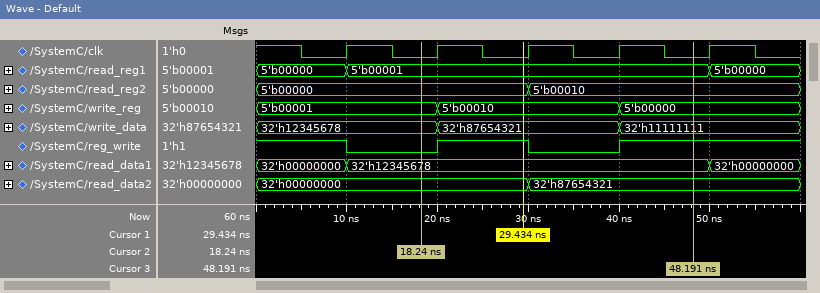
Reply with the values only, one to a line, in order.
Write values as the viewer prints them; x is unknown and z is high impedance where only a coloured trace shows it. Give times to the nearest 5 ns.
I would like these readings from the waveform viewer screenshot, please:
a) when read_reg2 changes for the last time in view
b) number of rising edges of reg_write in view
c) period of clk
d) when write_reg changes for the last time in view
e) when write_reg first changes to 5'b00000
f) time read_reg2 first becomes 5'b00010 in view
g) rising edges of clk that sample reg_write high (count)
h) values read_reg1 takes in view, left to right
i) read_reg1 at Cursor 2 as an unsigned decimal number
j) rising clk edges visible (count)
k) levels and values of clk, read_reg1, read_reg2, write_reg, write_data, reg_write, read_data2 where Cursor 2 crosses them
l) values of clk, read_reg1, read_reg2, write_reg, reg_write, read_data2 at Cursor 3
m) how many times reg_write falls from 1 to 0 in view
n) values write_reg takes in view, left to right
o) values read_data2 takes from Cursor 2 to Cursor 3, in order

30 ns
2
10 ns
40 ns
40 ns
30 ns
3
5'b00000, 5'b00001, 5'b00000
1
5
clk=0, read_reg1=5'b00001, read_reg2=5'b00000, write_reg=5'b00001, write_data=32'h12345678, reg_write=0, read_data2=32'h00000000
clk=0, read_reg1=5'b00001, read_reg2=5'b00010, write_reg=5'b00000, reg_write=1, read_data2=32'h87654321
2
5'b00001, 5'b00010, 5'b00000
32'h00000000, 32'h87654321
